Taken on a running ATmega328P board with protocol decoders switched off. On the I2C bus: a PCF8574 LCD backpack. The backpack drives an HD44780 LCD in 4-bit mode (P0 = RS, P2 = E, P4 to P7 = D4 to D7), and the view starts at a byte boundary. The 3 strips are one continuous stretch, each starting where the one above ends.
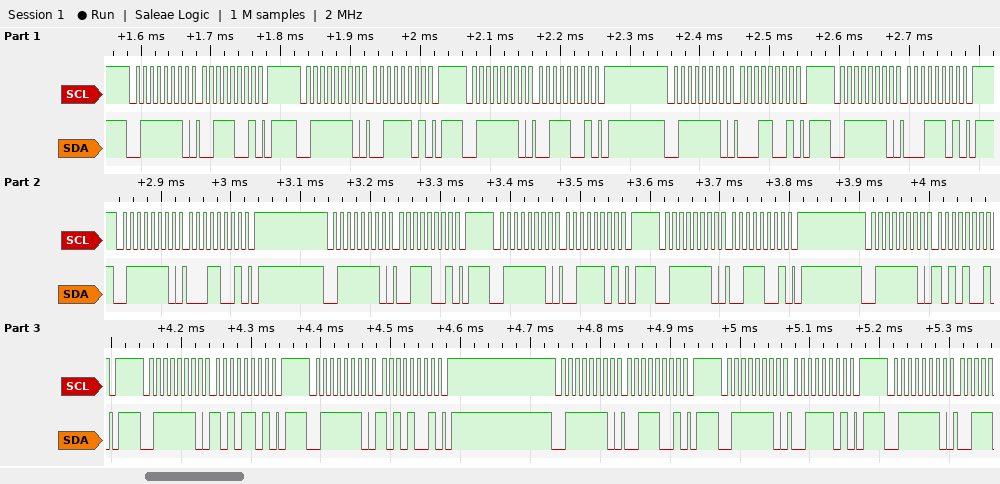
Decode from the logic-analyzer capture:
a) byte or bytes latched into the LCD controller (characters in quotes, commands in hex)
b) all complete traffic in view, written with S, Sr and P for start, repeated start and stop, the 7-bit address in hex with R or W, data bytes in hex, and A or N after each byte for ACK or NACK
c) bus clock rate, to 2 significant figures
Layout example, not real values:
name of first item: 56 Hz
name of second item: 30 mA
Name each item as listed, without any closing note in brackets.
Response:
byte or bytes latched into the LCD controller: '1' ':'
all complete traffic in view, written with S, Sr and P for start, repeated start and stop, the 7-bit address in hex with R or W, data bytes in hex, and A or N after each byte for ACK or NACK: S 3FW A 39 A P S 3FW A 3D A P S 3FW A 39 A P S 3FW A 19 A P S 3FW A 1D A P S 3FW A 19 A P S 3FW A 39 A P S 3FW A 3D A P S 3FW A 39 A P S 3FW A A9 A P S 3FW A AD A P S 3FW A A9 A P S 3FW A 39 A P S 3FW A 3D A P S 3FW A
bus clock rate, to 2 significant figures: 100 kHz
